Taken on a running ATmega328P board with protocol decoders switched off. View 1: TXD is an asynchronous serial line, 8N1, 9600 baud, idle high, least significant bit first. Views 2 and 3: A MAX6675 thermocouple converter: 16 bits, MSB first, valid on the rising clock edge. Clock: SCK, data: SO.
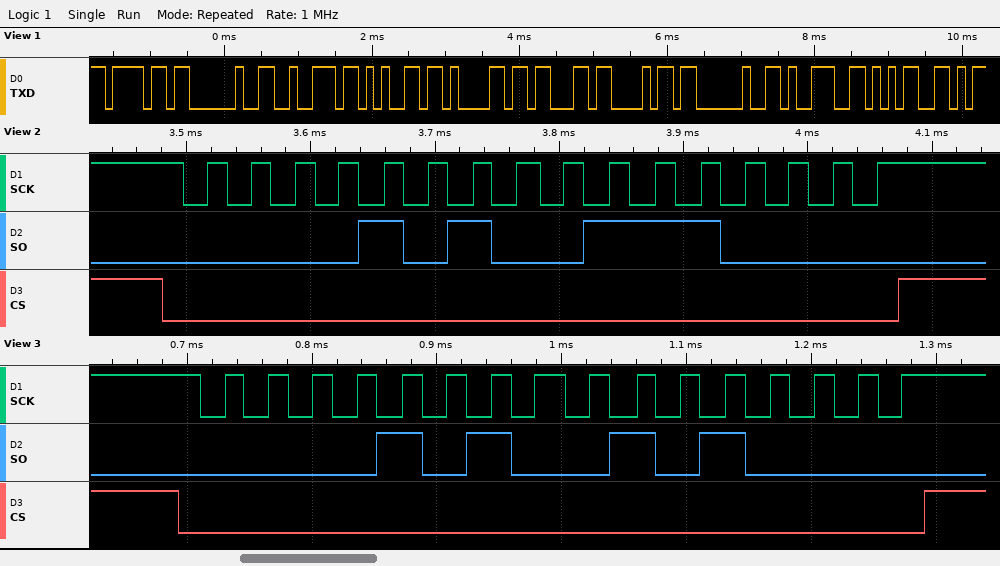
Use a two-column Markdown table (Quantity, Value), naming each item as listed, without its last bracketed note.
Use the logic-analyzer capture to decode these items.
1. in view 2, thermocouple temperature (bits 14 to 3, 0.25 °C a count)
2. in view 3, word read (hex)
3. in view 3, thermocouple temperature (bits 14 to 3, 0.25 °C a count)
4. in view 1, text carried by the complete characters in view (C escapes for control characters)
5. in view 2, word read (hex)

| Quantity | Value |
|---|---|
| in view 2, thermocouple temperature | 83.50 °C |
| in view 3, word read | 0x0A50 |
| in view 3, thermocouple temperature | 82.50 °C |
| in view 1, text carried by the complete characters in view | "o reach 95" |
| in view 2, word read | 0x0A70 |
